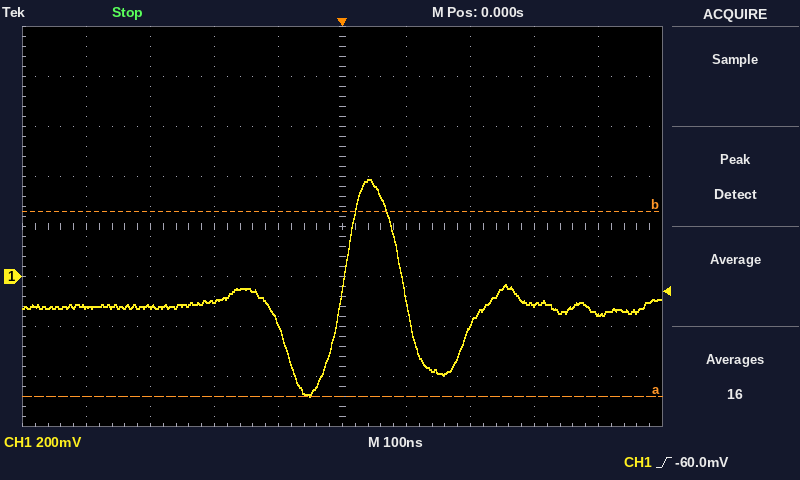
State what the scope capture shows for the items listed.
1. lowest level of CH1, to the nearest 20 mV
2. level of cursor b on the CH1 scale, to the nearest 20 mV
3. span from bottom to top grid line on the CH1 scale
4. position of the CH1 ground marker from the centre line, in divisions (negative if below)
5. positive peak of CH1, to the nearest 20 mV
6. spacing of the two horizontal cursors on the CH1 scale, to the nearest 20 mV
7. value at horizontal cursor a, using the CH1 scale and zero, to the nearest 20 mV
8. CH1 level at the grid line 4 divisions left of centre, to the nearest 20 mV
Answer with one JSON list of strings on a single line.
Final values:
["-480 mV", "260 mV", "1.6 V", "-1.0 div", "380 mV", "740 mV", "-480 mV", "-120 mV"]
